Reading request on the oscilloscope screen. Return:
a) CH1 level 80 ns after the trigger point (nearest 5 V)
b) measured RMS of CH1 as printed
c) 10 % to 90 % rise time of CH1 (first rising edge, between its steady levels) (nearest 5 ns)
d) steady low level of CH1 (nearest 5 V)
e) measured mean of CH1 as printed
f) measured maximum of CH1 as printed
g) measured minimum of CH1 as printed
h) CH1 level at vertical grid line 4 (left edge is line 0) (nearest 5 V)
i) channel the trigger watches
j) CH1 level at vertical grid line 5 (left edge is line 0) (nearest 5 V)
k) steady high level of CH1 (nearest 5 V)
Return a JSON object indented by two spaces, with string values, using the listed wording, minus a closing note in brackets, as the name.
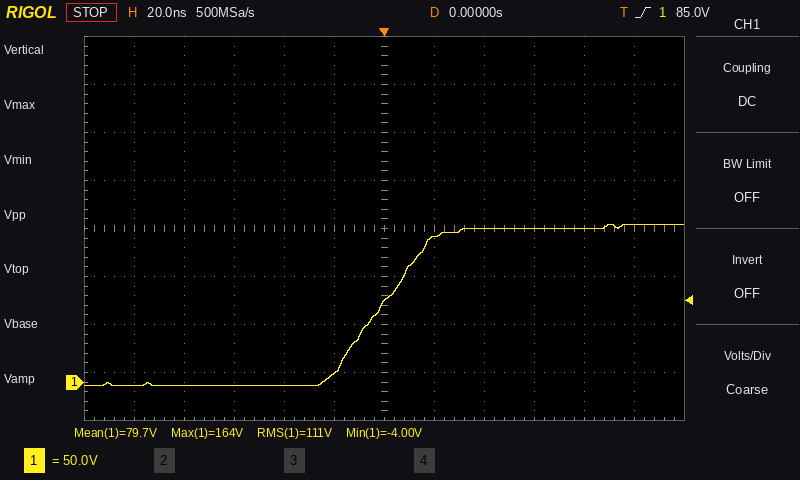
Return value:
{
  "CH1 level 80 ns after the trigger point": "160 V",
  "measured RMS of CH1 as printed": "111 V",
  "10 % to 90 % rise time of CH1 (first rising edge, between its steady levels)": "35 ns",
  "steady low level of CH1": "-5 V",
  "measured mean of CH1 as printed": "79.7 V",
  "measured maximum of CH1 as printed": "164 V",
  "measured minimum of CH1 as printed": "-4.00 V",
  "CH1 level at vertical grid line 4 (left edge is line 0)": "-5 V",
  "channel the trigger watches": "CH1",
  "CH1 level at vertical grid line 5 (left edge is line 0)": "10 V",
  "steady high level of CH1": "160 V"
}
